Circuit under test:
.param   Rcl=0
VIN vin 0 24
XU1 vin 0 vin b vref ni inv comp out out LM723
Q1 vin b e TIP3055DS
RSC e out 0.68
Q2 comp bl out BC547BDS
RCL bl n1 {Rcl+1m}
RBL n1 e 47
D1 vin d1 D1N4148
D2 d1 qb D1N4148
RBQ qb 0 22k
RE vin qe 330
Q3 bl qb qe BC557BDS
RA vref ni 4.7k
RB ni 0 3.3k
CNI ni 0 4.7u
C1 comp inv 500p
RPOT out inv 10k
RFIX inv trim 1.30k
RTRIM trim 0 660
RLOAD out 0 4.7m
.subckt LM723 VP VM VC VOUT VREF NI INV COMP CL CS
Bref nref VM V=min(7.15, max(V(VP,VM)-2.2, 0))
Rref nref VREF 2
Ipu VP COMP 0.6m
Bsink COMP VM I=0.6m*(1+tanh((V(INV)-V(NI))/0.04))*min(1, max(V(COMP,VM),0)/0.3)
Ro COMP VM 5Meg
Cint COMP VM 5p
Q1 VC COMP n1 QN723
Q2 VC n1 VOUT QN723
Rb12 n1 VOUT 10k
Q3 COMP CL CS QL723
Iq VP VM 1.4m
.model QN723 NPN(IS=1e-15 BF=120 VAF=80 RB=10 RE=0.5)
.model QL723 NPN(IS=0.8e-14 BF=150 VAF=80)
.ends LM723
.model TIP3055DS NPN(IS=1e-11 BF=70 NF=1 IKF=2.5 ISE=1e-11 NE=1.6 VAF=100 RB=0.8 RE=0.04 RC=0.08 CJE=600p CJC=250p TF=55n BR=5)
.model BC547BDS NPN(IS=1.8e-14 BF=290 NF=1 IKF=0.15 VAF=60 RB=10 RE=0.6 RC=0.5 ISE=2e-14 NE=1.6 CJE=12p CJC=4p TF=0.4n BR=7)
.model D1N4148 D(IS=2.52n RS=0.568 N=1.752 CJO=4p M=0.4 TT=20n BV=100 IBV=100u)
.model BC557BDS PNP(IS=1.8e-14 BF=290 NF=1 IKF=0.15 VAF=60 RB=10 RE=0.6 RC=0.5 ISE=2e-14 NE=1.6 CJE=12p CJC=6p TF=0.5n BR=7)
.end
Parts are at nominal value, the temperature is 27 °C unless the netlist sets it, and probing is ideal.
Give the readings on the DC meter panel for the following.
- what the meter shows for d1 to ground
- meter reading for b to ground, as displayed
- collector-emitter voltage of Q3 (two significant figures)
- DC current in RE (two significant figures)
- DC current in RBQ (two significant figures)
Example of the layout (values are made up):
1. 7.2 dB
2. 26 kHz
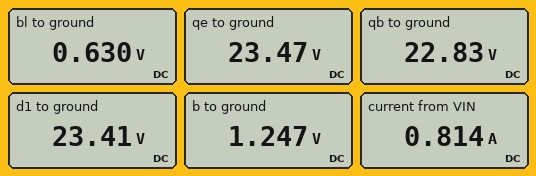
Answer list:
1. 23.41 V
2. 1.247 V
3. -23 V
4. 1.6 mA
5. 1.0 mA
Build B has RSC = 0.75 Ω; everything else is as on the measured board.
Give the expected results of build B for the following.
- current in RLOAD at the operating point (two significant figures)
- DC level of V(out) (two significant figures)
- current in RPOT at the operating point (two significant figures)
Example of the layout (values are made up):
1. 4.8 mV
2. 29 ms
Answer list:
1. 740 mA
2. 3.5 mV
3. 290 nA
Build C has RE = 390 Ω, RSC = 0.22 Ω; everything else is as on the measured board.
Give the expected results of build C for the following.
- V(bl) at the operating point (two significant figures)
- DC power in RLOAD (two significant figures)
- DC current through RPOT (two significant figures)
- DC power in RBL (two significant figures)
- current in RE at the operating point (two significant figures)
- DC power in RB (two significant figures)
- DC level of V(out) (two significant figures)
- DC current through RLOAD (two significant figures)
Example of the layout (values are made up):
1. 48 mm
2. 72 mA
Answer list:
1. 640 mV
2. 31 mW
3. 1.0 µA
4. 87 µW
5. 1.4 mA
6. 2.6 mW
7. 12 mV
8. 2.6 A
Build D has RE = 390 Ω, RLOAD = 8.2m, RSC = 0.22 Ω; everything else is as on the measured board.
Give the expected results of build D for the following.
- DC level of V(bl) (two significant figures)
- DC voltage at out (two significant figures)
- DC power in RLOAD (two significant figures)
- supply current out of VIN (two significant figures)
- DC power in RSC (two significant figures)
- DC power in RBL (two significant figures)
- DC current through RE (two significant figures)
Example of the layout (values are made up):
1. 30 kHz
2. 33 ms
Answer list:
1. 650 mV
2. 21 mV
3. 54 mW
4. 2.6 A
5. 1.4 W
6. 87 µW
7. 1.4 mA
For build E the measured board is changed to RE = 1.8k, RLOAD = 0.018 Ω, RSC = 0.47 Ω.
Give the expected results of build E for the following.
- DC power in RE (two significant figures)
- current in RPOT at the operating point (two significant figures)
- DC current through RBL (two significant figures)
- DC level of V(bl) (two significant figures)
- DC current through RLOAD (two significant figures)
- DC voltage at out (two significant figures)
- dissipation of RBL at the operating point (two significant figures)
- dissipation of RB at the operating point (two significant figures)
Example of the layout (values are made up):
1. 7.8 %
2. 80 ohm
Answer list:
1. 180 µW
2. 2.0 µA
3. 310 µA
4. 650 mV
5. 1.3 A
6. 23 mV
7. 4.6 µW
8. 2.6 mW
